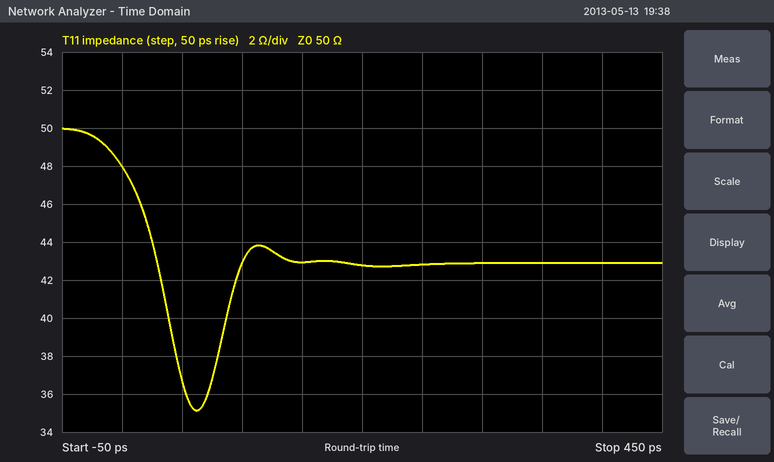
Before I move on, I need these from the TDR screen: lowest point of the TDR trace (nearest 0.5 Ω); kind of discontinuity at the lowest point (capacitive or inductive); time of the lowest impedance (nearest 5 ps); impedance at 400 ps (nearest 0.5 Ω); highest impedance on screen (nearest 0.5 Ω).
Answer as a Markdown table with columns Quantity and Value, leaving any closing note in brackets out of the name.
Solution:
| Quantity | Value |
|---|---|
| lowest point of the TDR trace | 35.0 Ω |
| kind of discontinuity at the lowest point | capacitive |
| time of the lowest impedance | 60 ps |
| impedance at 400 ps | 43.0 Ω |
| highest impedance on screen | 50.0 Ω |
